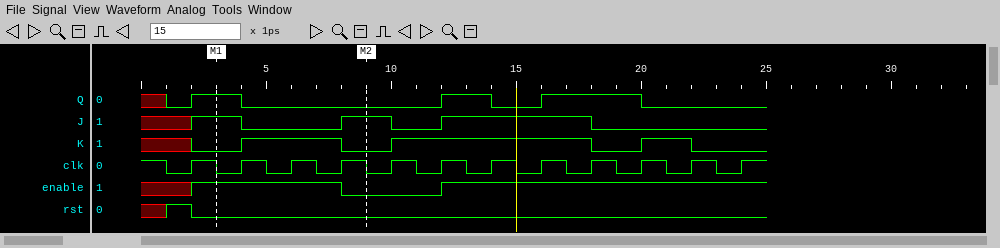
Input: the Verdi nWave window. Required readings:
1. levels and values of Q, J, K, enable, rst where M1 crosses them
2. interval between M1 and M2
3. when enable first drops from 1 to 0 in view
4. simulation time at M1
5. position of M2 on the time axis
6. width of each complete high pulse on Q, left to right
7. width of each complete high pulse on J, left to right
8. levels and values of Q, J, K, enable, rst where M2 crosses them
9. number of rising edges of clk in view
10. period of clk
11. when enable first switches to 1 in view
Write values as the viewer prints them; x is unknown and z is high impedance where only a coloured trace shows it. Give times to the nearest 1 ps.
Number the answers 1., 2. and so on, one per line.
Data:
1. Q=1, J=1, K=0, enable=1, rst=0
2. 6 ps
3. 8 ps
4. 3 ps
5. 9 ps
6. 2 ps, 2 ps, 4 ps
7. 2 ps, 6 ps
8. Q=0, J=1, K=0, enable=0, rst=0
9. 12
10. 2 ps
11. 2 ps
